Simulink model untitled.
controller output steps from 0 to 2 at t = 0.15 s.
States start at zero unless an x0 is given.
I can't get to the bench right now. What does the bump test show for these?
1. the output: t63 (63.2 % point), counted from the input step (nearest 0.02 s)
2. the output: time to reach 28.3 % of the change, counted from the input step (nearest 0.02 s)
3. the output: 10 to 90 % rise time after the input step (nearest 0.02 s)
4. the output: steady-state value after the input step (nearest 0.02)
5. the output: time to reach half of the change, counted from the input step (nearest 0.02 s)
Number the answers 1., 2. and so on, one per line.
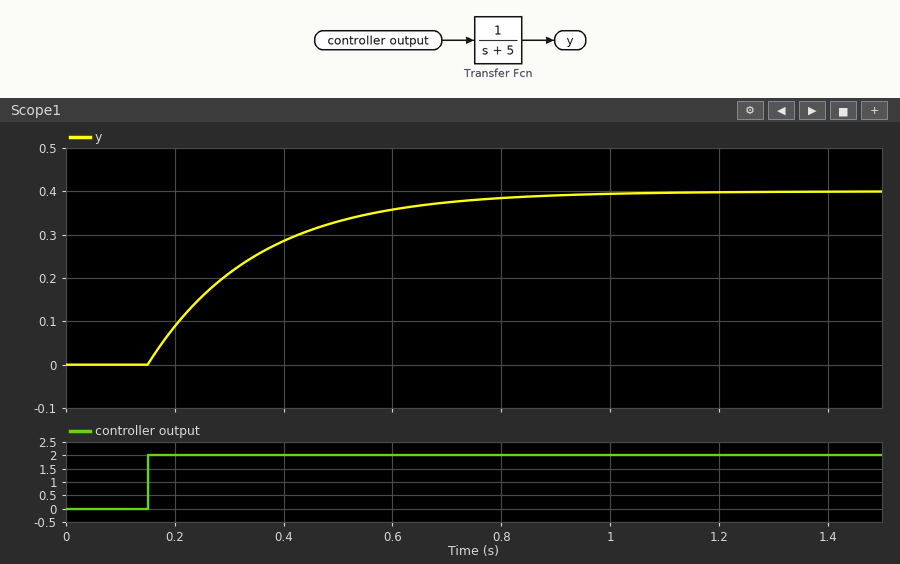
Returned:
1. 0.20 s
2. 0.06 s
3. 0.44 s
4. 0.40
5. 0.14 s
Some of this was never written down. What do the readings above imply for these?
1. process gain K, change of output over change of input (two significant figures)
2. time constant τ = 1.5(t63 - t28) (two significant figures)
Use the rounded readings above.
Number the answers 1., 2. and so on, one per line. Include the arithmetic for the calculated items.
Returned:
1. (0.4 - 0) / 2 = 0.20
2. 1.5 × (0.2 - 0.06) = 0.21 s
